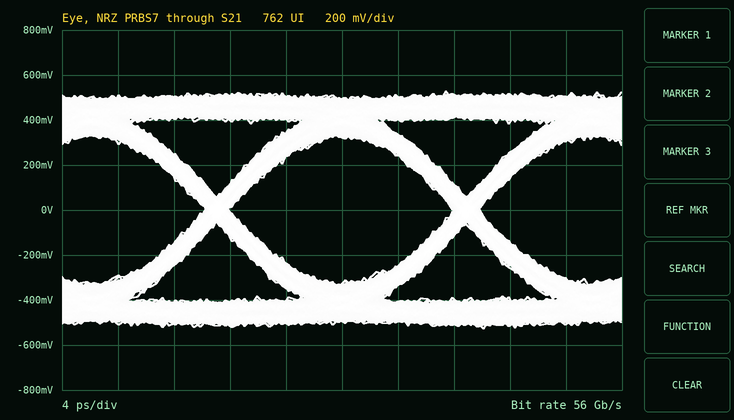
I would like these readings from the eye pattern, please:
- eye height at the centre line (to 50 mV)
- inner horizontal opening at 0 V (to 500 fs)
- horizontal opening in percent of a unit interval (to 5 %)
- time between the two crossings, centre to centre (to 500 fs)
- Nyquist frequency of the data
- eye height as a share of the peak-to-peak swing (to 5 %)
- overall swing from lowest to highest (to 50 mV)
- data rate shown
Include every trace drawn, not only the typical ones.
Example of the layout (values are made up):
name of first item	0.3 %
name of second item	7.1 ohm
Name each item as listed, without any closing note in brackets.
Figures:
eye height at the centre line	650 mV
inner horizontal opening at 0 V	16.0 ps
horizontal opening in percent of a unit interval	90 %
time between the two crossings, centre to centre	18.0 ps
Nyquist frequency of the data	28 GHz
eye height as a share of the peak-to-peak swing	60 %
overall swing from lowest to highest	1.05 V
data rate shown	56 Gb/s
